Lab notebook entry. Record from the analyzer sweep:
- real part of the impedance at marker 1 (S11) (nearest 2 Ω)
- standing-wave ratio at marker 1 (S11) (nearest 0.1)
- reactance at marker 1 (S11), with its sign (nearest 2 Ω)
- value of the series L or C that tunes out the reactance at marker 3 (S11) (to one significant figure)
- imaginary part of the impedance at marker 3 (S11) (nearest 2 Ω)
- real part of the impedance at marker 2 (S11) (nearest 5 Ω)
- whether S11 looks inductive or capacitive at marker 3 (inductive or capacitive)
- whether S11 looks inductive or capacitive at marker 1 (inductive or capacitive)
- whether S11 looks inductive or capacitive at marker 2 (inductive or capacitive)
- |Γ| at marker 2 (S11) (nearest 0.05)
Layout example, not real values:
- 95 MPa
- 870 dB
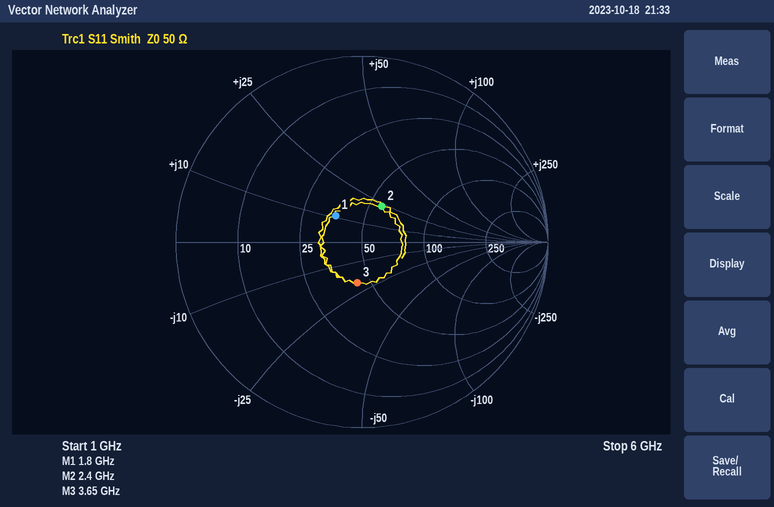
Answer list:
- 36 Ω
- 1.5
- +10 Ω
- 900 pH
- -20 Ω
- 55 Ω
- capacitive
- inductive
- inductive
- 0.20
